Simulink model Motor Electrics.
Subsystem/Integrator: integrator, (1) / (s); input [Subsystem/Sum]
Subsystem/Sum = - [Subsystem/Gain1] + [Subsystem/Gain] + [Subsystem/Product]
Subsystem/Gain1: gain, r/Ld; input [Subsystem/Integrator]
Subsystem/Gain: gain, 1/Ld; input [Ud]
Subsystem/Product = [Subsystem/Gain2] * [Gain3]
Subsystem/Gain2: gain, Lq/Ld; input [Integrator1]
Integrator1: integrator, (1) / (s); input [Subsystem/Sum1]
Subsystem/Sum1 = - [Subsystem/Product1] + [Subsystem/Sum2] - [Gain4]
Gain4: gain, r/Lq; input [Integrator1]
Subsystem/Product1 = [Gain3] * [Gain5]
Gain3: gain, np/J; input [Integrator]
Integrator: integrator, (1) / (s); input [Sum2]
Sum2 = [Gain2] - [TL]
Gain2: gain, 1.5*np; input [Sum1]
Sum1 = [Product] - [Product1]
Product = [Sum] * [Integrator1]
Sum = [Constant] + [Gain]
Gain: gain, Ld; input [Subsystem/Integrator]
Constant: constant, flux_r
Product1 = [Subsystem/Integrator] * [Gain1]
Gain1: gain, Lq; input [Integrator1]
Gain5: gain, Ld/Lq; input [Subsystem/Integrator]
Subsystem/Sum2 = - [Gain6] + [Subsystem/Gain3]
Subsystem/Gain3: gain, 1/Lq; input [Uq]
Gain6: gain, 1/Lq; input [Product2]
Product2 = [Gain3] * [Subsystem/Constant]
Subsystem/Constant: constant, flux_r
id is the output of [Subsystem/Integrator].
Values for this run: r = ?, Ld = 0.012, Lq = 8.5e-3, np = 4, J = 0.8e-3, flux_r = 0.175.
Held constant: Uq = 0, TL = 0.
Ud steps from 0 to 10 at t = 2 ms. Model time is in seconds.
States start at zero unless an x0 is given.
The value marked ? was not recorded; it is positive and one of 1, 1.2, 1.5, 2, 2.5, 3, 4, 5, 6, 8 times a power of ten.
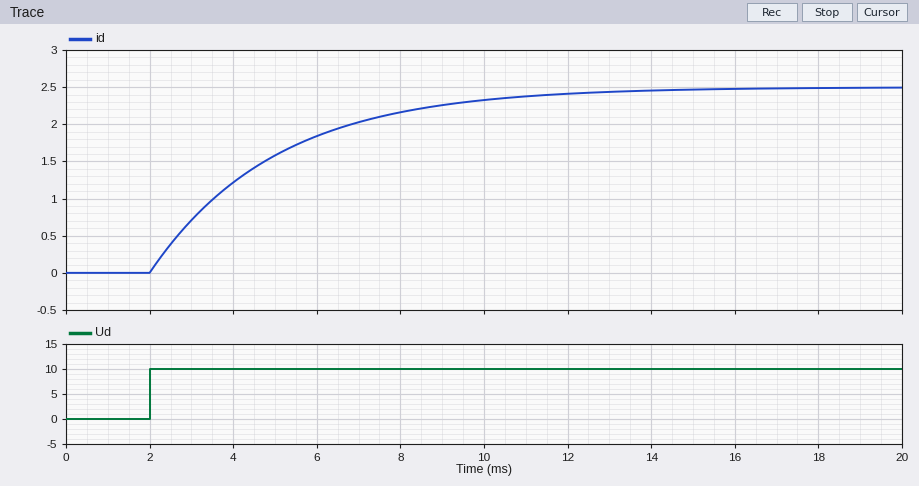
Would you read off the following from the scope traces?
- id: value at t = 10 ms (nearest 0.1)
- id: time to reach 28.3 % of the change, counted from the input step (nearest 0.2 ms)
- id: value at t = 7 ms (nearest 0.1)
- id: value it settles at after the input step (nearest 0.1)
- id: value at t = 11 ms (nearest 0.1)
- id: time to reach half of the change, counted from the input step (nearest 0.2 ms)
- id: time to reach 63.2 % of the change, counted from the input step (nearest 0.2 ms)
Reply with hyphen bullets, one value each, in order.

- 2.3
- 1.0 ms
- 2.0
- 2.5
- 2.4
- 2.0 ms
- 3.0 ms
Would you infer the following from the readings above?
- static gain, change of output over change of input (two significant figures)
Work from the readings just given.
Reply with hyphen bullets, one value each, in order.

- 0.25
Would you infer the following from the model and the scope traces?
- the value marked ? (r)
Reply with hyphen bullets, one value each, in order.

- 4
